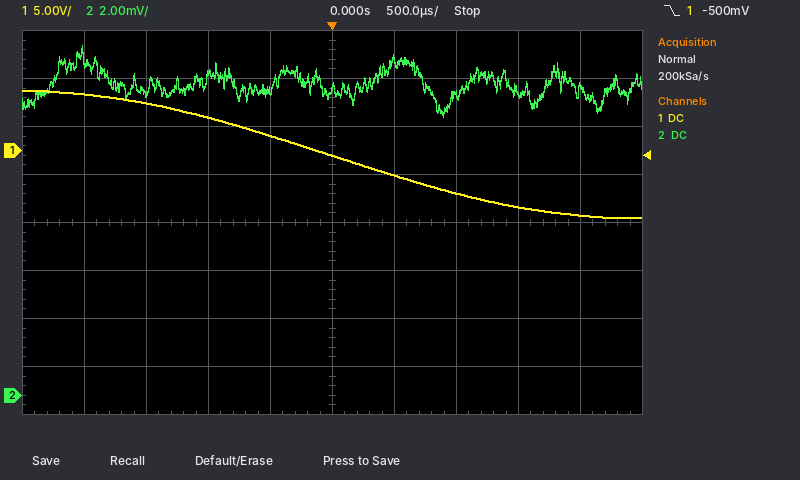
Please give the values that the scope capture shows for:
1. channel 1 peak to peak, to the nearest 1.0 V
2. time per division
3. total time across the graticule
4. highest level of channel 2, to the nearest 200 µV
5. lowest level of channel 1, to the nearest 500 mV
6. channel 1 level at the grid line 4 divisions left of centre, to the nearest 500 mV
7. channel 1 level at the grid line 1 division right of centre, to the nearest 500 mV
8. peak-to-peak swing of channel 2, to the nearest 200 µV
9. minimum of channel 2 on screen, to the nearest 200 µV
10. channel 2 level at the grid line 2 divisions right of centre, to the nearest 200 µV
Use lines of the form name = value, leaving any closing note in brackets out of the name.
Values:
channel 1 peak to peak, to the nearest 1.0 V = 13.0 V
time per division = 500 µs
total time across the graticule = 5 ms
highest level of channel 2, to the nearest 200 µV = 14.6 mV
lowest level of channel 1, to the nearest 500 mV = -7.0 V
channel 1 level at the grid line 4 divisions left of centre, to the nearest 500 mV = 6.0 V
channel 1 level at the grid line 1 division right of centre, to the nearest 500 mV = -2.5 V
peak-to-peak swing of channel 2, to the nearest 200 µV = 3.0 mV
minimum of channel 2 on screen, to the nearest 200 µV = 11.6 mV
channel 2 level at the grid line 2 divisions right of centre, to the nearest 200 µV = 12.6 mV
